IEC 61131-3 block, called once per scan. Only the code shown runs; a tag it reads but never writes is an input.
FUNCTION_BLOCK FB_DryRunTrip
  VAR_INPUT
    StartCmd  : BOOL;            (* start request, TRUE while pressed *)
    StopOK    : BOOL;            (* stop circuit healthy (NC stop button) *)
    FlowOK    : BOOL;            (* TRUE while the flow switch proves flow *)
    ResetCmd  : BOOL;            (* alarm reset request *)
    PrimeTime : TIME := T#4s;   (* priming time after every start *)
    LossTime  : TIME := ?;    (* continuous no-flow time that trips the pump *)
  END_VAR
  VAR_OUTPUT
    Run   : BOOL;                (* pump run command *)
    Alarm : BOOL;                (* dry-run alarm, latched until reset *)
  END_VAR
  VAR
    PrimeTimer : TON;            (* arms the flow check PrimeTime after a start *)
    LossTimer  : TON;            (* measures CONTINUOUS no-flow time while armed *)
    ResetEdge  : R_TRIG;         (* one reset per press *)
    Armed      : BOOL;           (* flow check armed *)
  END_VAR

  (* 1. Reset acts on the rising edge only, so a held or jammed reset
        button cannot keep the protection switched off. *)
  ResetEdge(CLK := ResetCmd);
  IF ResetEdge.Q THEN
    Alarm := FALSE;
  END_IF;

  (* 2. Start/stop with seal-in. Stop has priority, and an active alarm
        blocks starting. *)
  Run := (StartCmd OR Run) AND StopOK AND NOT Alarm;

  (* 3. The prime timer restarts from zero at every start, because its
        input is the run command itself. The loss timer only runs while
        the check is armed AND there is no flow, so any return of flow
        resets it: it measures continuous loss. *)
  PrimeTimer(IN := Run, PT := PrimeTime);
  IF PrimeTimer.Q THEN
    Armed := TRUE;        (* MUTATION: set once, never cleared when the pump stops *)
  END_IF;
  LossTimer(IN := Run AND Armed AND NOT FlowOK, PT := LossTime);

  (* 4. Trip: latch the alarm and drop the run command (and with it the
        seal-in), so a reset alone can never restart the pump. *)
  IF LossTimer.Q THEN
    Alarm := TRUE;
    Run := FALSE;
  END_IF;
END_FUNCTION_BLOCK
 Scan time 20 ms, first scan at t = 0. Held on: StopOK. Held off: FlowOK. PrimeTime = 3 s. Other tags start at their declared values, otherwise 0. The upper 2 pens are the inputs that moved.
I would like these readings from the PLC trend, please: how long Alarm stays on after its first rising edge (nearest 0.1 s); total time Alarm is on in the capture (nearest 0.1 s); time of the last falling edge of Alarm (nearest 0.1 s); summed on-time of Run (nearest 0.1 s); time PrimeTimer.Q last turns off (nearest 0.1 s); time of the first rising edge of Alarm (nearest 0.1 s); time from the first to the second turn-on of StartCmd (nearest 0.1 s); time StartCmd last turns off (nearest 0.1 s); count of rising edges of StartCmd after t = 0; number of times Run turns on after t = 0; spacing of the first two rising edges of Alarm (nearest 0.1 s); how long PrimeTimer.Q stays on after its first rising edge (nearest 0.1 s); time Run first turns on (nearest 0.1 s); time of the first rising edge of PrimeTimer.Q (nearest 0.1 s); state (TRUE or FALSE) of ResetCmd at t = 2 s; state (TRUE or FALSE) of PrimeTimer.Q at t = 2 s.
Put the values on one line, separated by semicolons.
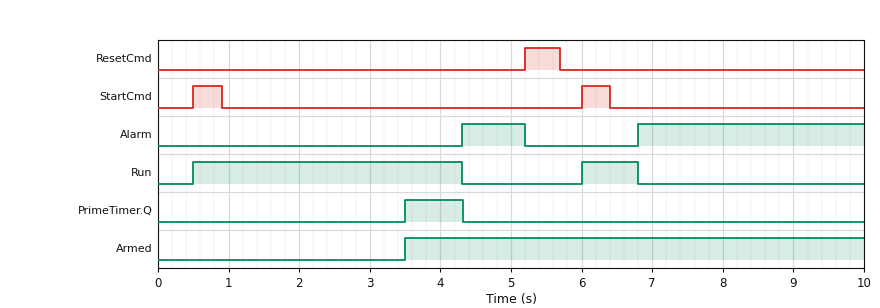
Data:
0.9 s; 4.1 s; 5.2 s; 4.6 s; 4.3 s; 4.3 s; 5.5 s; 6.4 s; 2; 2; 2.5 s; 0.8 s; 0.5 s; 3.5 s; FALSE; FALSE
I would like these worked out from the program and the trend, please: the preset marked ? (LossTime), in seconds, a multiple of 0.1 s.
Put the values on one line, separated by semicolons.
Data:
0.8 s
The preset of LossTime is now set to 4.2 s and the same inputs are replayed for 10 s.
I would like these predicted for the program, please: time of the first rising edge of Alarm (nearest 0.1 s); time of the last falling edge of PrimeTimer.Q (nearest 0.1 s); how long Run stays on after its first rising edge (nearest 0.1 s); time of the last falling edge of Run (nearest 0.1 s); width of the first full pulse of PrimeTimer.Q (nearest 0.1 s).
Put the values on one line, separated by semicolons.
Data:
7.7 s; 7.7 s; 7.2 s; 7.7 s; 4.2 s
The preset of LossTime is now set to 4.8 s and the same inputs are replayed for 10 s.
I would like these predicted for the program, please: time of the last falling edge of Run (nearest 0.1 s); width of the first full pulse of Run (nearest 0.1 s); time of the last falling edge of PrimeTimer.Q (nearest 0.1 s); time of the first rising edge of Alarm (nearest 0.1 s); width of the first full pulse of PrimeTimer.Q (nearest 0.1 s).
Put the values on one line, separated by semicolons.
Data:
8.3 s; 7.8 s; 8.3 s; 8.3 s; 4.8 s
